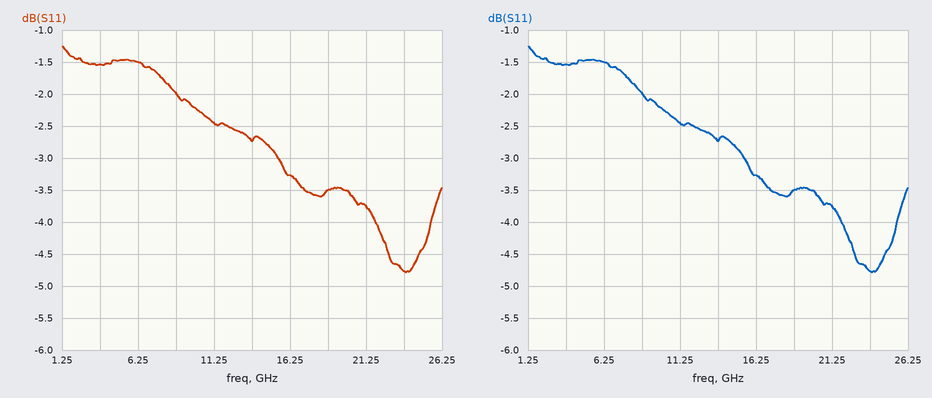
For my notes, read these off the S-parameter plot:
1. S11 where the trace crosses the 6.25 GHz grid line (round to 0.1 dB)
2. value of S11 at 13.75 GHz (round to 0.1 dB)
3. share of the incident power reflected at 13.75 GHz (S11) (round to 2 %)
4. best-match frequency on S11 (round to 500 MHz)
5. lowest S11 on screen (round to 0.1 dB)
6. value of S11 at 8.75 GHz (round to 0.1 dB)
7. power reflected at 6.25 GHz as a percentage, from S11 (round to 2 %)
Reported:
-1.5 dB
-2.7 dB
54 %
24.0 GHz
-4.8 dB
-2.0 dB
70 %
